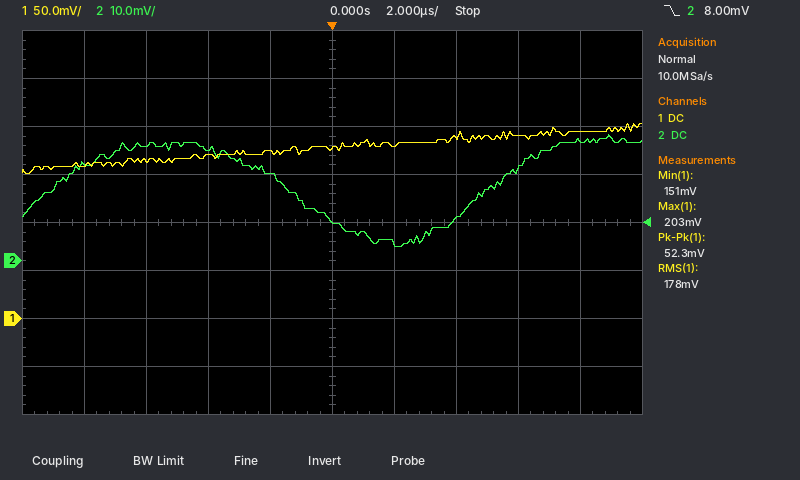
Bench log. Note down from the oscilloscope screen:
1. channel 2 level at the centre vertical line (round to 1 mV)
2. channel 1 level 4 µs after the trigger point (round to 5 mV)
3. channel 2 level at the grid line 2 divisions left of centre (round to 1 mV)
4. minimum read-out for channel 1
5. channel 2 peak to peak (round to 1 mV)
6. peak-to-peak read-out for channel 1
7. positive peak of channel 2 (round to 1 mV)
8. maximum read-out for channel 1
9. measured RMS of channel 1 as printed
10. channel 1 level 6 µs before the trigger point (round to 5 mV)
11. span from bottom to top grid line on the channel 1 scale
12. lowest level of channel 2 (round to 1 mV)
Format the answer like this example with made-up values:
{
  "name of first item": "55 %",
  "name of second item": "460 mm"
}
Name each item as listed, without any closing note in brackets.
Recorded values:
{
  "channel 2 level at the centre vertical line": "8 mV",
  "channel 1 level 4 µs after the trigger point": "190 mV",
  "channel 2 level at the grid line 2 divisions left of centre": "23 mV",
  "minimum read-out for channel 1": "151 mV",
  "channel 2 peak to peak": "23 mV",
  "peak-to-peak read-out for channel 1": "52.3 mV",
  "positive peak of channel 2": "26 mV",
  "maximum read-out for channel 1": "203 mV",
  "measured RMS of channel 1 as printed": "178 mV",
  "channel 1 level 6 µs before the trigger point": "165 mV",
  "span from bottom to top grid line on the channel 1 scale": "400 mV",
  "lowest level of channel 2": "3 mV"
}
